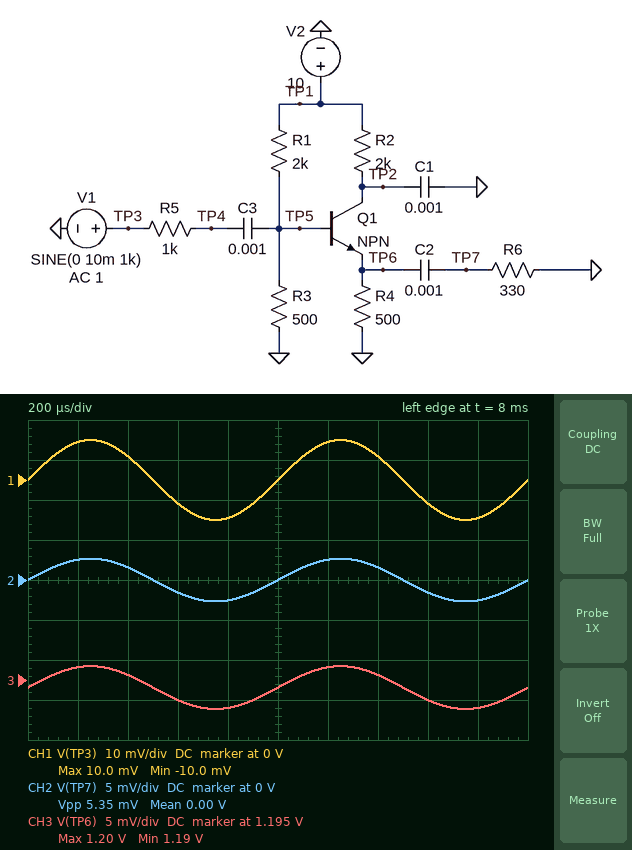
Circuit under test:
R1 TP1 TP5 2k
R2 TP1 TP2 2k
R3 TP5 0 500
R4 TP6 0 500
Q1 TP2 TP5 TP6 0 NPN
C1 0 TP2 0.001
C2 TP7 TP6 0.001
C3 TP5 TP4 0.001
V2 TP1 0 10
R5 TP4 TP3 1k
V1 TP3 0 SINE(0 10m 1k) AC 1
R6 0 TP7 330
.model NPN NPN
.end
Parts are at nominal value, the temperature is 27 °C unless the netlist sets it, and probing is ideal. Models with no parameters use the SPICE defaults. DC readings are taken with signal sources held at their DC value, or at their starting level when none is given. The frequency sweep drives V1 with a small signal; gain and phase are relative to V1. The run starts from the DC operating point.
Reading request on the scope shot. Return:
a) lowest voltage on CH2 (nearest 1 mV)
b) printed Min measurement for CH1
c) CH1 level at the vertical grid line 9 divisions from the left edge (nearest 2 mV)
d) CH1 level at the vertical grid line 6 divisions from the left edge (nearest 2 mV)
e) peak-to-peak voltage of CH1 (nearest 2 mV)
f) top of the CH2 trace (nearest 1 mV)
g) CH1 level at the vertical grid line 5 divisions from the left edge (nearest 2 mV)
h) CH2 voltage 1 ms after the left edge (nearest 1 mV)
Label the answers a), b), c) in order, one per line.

a) -3 mV
b) -10.0 mV
c) -10 mV
d) 10 mV
e) 20 mV
f) 3 mV
g) 0 V
h) 0 V
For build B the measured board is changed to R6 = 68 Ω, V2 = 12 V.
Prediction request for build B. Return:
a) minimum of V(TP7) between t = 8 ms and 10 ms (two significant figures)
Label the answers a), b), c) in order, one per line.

a) -2.4 mV
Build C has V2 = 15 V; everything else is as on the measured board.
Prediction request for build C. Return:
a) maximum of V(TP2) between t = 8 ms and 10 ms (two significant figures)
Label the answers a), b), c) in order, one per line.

a) 6.4 V
